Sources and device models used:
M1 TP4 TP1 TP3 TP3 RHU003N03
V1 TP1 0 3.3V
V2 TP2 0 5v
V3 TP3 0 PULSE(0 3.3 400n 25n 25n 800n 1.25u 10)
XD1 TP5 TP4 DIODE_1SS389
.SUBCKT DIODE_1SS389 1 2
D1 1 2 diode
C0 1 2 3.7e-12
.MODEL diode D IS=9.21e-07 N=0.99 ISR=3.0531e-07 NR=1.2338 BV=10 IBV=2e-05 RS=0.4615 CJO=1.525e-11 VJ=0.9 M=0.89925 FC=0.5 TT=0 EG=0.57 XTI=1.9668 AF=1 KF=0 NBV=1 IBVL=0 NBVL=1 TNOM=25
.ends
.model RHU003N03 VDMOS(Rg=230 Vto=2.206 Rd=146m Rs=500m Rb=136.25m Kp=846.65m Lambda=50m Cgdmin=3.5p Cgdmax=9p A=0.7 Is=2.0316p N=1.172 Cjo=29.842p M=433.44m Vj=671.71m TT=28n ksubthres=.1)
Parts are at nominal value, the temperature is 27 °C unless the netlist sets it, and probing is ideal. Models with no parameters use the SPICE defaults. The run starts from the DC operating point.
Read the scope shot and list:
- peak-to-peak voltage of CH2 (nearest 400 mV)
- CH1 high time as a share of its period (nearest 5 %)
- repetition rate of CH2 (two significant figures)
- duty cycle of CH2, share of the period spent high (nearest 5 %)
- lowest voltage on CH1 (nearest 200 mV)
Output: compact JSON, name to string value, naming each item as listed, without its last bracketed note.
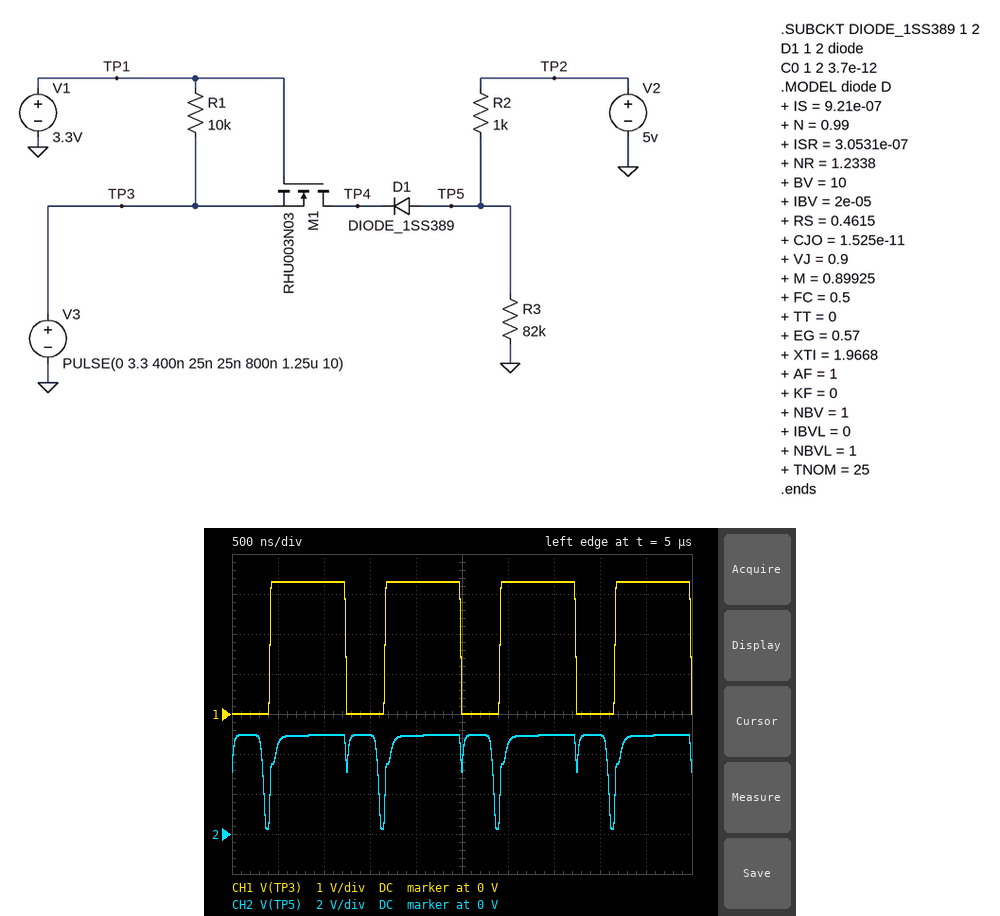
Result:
{"peak-to-peak voltage of CH2": "4.8 V", "CH1 high time as a share of its period": "65 %", "repetition rate of CH2": "800 kHz", "duty cycle of CH2, share of the period spent high": "95 %", "lowest voltage on CH1": "0 V"}
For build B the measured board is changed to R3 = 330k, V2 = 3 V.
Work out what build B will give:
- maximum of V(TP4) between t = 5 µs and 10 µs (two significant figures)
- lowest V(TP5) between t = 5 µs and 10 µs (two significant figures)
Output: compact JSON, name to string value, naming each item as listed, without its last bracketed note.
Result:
{"maximum of V(TP4) between t = 5 µs and 10 µs": "3.3 V", "lowest V(TP5) between t = 5 µs and 10 µs": "220 mV"}
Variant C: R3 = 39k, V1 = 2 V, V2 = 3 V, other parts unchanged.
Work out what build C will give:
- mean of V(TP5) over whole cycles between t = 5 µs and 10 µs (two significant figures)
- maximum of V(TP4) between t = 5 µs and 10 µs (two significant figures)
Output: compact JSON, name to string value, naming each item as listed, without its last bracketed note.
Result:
{"mean of V(TP5) over whole cycles between t = 5 µs and 10 µs": "2.9 V", "maximum of V(TP4) between t = 5 µs and 10 µs": "5.4 V"}
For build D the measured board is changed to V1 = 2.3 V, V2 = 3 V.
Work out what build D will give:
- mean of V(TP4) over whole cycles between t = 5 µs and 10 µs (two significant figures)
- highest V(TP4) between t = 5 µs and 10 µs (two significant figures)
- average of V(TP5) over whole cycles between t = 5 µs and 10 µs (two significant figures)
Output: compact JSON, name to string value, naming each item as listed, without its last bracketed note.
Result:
{"mean of V(TP4) over whole cycles between t = 5 µs and 10 µs": "4.3 V", "highest V(TP4) between t = 5 µs and 10 µs": "5.5 V", "average of V(TP5) over whole cycles between t = 5 µs and 10 µs": "3.0 V"}
